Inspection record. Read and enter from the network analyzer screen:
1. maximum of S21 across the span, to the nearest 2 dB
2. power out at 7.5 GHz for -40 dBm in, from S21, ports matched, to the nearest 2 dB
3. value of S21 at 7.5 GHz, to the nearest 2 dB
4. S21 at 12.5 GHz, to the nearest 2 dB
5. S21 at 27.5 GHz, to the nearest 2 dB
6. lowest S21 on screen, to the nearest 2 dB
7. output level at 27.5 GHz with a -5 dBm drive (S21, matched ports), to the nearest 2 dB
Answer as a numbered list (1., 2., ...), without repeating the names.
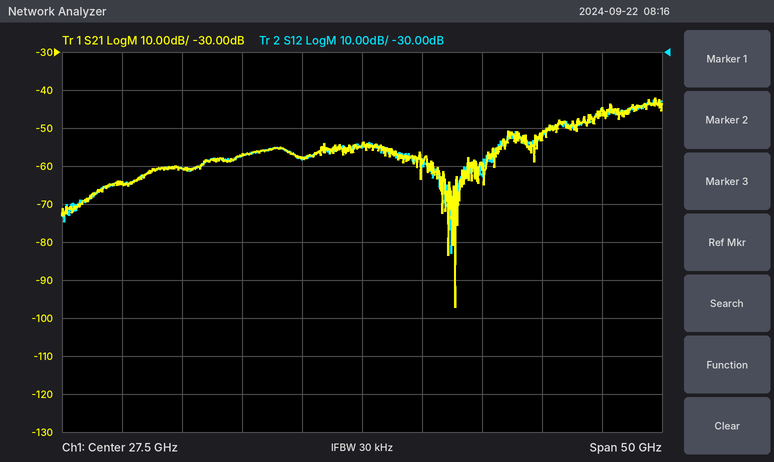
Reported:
1. -42 dB
2. -104 dBm
3. -64 dB
4. -60 dB
5. -54 dB
6. -98 dB
7. -60 dBm
